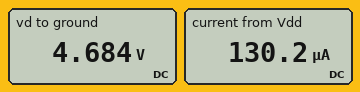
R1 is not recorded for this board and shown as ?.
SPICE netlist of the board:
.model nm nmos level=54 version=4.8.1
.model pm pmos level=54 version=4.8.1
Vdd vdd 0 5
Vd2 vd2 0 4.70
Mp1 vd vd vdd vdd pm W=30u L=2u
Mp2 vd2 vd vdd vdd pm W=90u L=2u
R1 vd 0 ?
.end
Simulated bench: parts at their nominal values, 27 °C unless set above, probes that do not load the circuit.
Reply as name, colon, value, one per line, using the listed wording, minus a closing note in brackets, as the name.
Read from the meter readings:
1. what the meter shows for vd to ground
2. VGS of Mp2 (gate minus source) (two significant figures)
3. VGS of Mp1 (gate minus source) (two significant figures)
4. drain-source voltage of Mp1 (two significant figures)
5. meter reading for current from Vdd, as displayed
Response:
what the meter shows for vd to ground: 4.684 V
VGS of Mp2 (gate minus source): -320 mV
VGS of Mp1 (gate minus source): -320 mV
drain-source voltage of Mp1: -320 mV
meter reading for current from Vdd, as displayed: 130.2 µA
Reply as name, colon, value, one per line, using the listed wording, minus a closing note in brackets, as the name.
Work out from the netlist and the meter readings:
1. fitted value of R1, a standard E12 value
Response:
fitted value of R1, a standard E12 value: 150 kΩ
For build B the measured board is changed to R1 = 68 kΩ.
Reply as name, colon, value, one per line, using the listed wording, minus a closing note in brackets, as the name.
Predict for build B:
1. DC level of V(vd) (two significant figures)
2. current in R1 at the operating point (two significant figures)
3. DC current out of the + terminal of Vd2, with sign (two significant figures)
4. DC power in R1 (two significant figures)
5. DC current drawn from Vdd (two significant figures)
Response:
DC level of V(vd): 4.6 V
current in R1 at the operating point: 68 µA
DC current out of the + terminal of Vd2, with sign: -210 µA
DC power in R1: 310 µW
DC current drawn from Vdd: 280 µA
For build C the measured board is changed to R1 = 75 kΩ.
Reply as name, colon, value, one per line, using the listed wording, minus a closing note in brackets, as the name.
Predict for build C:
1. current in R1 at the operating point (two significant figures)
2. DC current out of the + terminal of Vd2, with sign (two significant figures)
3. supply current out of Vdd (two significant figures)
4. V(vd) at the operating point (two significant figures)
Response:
current in R1 at the operating point: 62 µA
DC current out of the + terminal of Vd2, with sign: -190 µA
supply current out of Vdd: 250 µA
V(vd) at the operating point: 4.6 V
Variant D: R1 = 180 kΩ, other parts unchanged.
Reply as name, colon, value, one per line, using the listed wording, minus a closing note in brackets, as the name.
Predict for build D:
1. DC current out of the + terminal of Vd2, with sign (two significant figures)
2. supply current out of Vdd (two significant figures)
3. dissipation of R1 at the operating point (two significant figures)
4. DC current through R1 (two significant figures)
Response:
DC current out of the + terminal of Vd2, with sign: -83 µA
supply current out of Vdd: 110 µA
dissipation of R1 at the operating point: 120 µW
DC current through R1: 26 µA
